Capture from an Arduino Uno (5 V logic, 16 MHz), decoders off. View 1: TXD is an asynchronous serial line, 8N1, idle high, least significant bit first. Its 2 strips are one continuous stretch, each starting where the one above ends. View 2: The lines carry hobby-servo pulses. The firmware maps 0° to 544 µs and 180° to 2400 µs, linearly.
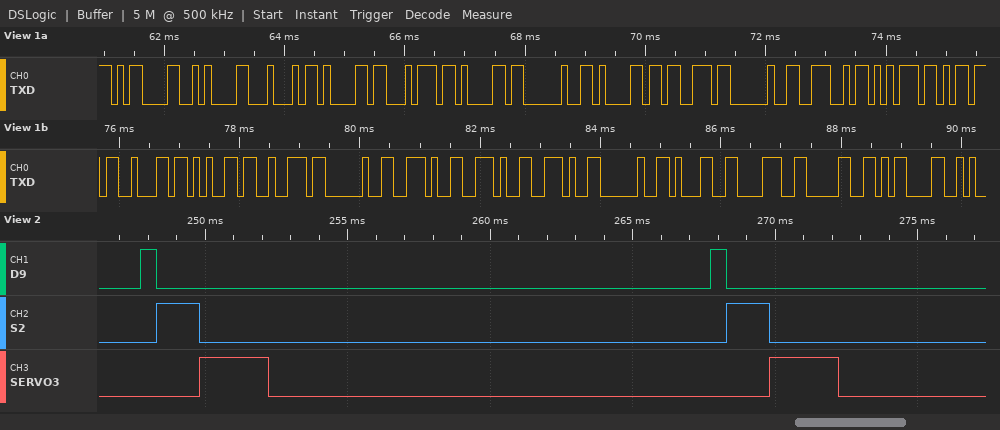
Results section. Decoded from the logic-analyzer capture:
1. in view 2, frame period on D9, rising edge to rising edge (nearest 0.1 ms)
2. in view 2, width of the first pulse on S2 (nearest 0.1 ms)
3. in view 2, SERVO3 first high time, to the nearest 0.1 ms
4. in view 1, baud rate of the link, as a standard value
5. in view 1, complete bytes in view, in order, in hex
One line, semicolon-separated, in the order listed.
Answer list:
20.0 ms; 1.5 ms; 2.4 ms; 9600 baud; 0D 0A 44 61 74 61 20 61 73 20 4E 75 6D 62 65 72 20 2E 2E 2E 20 31 38 30 0D
